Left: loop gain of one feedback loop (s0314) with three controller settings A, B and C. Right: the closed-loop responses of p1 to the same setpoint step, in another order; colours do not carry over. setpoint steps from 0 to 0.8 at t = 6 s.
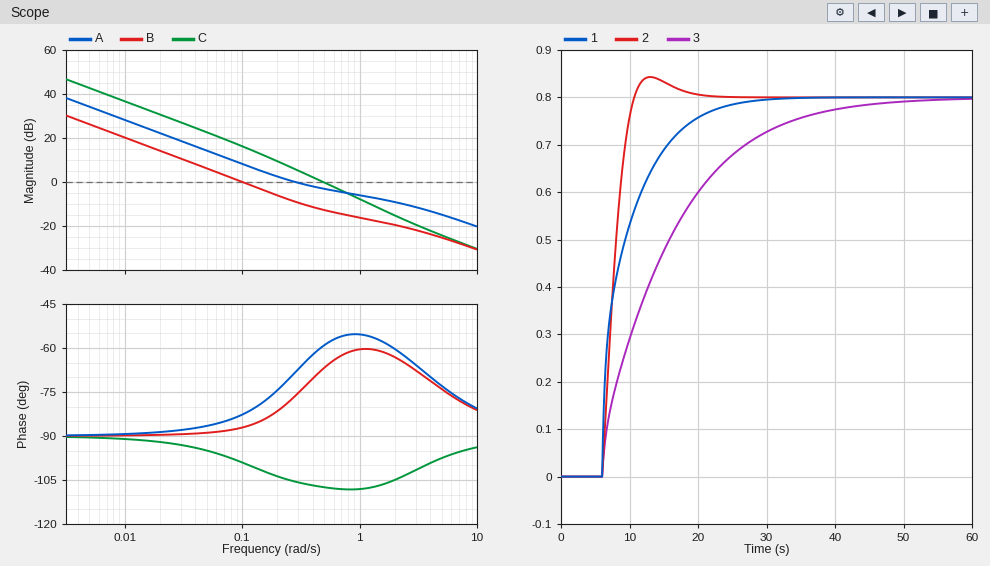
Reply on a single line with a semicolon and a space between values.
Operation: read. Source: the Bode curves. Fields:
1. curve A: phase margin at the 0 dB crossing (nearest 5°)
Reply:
110°
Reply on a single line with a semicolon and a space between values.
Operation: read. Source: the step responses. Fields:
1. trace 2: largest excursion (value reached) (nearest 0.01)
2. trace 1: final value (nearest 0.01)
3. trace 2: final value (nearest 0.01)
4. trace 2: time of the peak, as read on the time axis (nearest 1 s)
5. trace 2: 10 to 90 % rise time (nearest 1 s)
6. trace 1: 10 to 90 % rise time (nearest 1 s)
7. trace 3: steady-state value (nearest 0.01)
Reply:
0.84; 0.80; 0.80; 13 s; 3 s; 11 s; 0.80
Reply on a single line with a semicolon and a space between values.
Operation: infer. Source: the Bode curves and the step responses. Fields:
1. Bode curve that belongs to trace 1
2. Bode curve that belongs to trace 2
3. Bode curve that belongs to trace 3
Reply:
A; C; B
